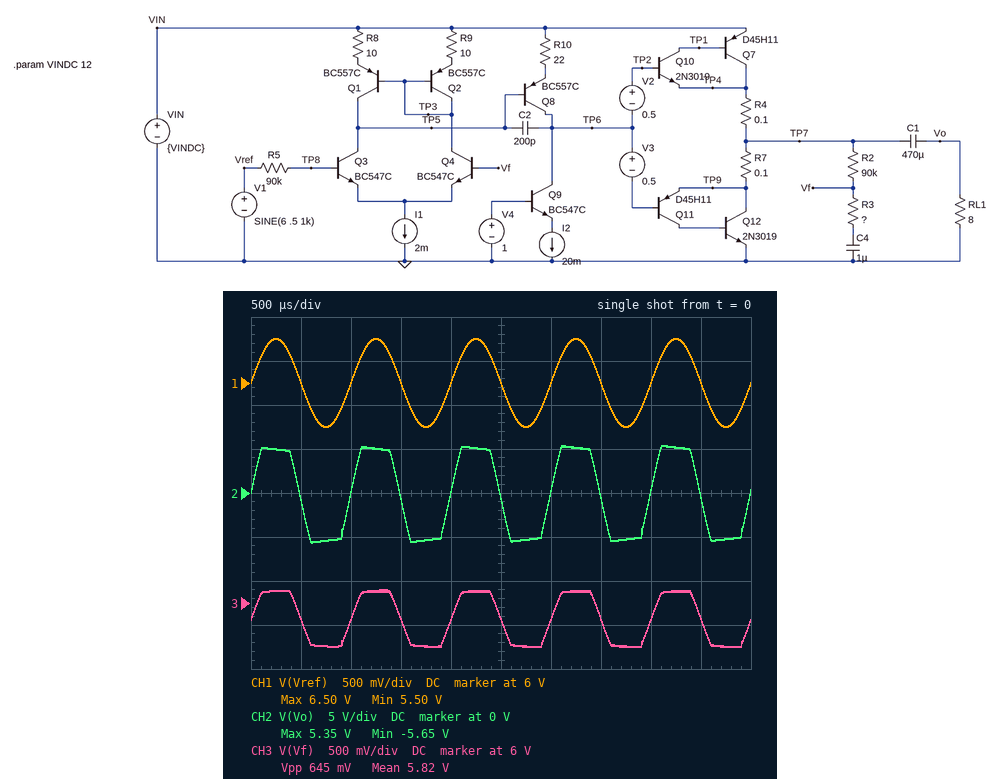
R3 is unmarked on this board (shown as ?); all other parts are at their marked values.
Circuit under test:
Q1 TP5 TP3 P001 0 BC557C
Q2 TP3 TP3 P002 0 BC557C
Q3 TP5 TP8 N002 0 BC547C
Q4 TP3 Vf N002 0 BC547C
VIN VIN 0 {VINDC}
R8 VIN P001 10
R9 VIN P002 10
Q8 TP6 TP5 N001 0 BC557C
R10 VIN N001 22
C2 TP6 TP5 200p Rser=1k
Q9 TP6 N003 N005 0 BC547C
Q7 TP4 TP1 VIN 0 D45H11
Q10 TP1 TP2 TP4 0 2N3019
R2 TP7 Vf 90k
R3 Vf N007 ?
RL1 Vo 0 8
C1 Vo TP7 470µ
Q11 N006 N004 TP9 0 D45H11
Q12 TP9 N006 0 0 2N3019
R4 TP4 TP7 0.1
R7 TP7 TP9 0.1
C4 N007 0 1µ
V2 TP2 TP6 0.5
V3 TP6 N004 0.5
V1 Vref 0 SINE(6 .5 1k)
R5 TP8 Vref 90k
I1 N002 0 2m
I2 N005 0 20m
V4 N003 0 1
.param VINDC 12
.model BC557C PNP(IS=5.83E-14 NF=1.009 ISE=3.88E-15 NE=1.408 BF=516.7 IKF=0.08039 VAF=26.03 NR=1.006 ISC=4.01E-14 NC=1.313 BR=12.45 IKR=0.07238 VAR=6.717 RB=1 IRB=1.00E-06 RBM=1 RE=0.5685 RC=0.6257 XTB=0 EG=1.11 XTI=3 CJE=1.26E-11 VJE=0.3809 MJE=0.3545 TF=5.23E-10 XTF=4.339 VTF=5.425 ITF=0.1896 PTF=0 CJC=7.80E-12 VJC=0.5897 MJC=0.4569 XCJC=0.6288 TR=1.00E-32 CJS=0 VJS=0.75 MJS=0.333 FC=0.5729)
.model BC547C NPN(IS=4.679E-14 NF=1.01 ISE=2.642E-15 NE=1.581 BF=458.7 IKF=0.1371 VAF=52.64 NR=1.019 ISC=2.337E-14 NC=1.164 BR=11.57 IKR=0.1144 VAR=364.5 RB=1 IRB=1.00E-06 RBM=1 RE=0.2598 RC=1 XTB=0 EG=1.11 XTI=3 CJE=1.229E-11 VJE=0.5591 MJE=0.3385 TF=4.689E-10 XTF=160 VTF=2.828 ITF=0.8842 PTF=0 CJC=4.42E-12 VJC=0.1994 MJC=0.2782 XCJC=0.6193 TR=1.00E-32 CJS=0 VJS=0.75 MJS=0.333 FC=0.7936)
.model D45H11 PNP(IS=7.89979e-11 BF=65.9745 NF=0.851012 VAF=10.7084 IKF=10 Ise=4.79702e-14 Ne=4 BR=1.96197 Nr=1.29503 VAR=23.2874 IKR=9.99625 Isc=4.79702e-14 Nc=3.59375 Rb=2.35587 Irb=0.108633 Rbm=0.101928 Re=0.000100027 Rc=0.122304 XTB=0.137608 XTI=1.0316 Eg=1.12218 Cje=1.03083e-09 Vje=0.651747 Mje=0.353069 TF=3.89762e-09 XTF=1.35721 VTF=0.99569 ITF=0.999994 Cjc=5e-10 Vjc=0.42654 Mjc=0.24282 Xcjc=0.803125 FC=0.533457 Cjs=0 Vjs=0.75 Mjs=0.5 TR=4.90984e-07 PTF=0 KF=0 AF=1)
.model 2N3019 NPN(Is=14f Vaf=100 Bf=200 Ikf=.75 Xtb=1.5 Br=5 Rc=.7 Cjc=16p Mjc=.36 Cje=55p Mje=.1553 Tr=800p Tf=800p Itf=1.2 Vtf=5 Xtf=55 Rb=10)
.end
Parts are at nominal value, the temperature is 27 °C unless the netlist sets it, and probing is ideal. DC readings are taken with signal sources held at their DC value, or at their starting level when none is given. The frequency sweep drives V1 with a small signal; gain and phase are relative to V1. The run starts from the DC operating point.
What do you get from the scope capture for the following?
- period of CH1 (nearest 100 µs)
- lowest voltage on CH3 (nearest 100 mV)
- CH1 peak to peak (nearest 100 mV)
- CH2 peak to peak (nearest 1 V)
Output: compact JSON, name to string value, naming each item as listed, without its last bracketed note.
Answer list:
{"period of CH1": "1.0 ms", "lowest voltage on CH3": "5.5 V", "CH1 peak to peak": "1.0 V", "CH2 peak to peak": "11 V"}
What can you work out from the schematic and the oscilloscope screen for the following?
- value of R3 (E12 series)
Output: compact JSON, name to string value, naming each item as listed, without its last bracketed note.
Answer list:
{"value of R3": "5.6 kΩ"}
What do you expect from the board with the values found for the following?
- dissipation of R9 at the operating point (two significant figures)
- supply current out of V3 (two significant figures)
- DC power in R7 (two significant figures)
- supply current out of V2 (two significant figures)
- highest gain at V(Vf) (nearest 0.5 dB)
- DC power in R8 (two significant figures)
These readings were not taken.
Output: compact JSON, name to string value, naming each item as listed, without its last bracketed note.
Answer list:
{"dissipation of R9 at the operating point": "9.4 µW", "supply current out of V3": "5.3 µA", "DC power in R7": "900 µW", "supply current out of V2": "4.6 µA", "highest gain at V(Vf)": "0 dB", "DC power in R8": "9.7 µW"}
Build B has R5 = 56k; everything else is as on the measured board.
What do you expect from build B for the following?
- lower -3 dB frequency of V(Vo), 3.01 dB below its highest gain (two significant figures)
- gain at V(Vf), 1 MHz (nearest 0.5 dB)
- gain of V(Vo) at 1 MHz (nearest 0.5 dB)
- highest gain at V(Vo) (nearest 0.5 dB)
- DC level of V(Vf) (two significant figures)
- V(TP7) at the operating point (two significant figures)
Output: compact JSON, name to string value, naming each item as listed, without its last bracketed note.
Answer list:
{"lower -3 dB frequency of V(Vo), 3.01 dB below its highest gain": "58 Hz", "gain at V(Vf), 1 MHz": "-13.5 dB", "gain of V(Vo) at 1 MHz": "12.5 dB", "highest gain at V(Vo)": "25.0 dB", "DC level of V(Vf)": "5.9 V", "V(TP7) at the operating point": "6.1 V"}
